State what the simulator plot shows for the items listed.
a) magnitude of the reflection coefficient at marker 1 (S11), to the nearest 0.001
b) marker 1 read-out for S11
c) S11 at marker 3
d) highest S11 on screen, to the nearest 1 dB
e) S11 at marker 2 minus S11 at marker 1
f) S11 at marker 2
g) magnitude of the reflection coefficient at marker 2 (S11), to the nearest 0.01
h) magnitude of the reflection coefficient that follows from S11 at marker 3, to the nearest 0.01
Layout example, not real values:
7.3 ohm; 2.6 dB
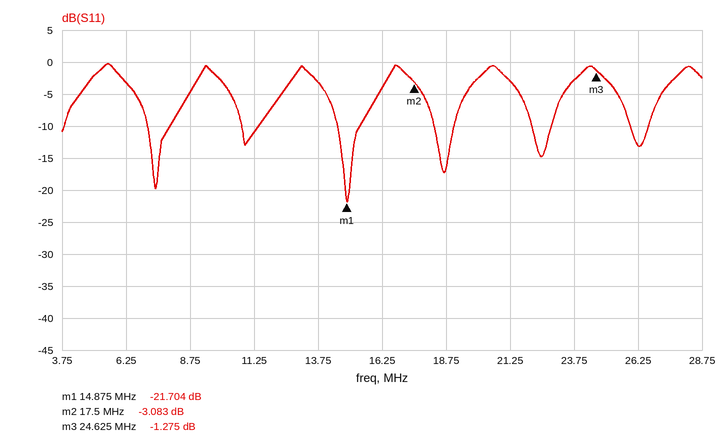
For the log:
0.082; -21.704 dB; -1.275 dB; 0 dB; 18.621 dB; -3.083 dB; 0.70; 0.86
